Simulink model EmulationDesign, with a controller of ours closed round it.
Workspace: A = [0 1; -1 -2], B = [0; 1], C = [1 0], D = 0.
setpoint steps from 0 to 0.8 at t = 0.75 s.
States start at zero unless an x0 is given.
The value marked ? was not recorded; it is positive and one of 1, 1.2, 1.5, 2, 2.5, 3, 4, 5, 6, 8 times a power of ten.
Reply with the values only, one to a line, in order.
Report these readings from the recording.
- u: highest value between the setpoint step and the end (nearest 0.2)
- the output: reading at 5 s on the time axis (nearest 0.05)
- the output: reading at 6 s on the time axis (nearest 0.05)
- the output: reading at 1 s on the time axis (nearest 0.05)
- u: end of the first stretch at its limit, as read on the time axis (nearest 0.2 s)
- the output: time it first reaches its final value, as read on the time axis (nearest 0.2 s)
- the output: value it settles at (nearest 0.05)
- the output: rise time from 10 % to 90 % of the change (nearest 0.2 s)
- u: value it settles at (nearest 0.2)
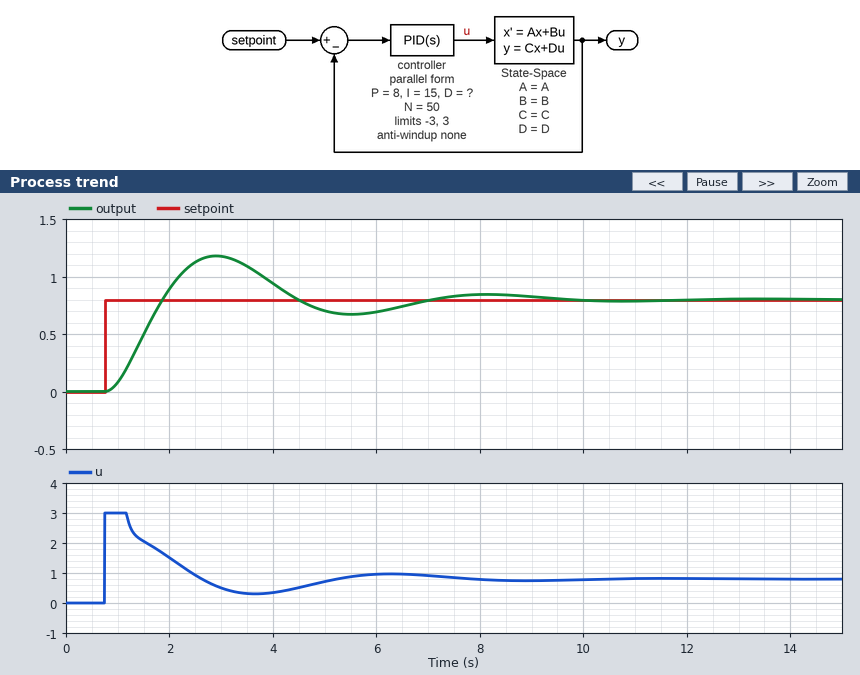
3.0
0.70
0.70
0.10
1.2 s
1.8 s
0.80
0.8 s
0.8
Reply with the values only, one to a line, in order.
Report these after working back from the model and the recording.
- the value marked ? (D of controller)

8
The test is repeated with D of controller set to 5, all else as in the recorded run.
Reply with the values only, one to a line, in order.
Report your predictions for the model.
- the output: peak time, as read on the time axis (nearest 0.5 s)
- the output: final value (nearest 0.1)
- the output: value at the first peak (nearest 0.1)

2.5 s
0.8
1.2
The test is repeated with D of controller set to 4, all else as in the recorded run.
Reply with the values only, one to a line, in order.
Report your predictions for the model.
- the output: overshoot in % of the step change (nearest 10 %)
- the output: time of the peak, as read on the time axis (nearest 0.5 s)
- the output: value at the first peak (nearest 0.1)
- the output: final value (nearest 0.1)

60 %
2.5 s
1.3
0.8
